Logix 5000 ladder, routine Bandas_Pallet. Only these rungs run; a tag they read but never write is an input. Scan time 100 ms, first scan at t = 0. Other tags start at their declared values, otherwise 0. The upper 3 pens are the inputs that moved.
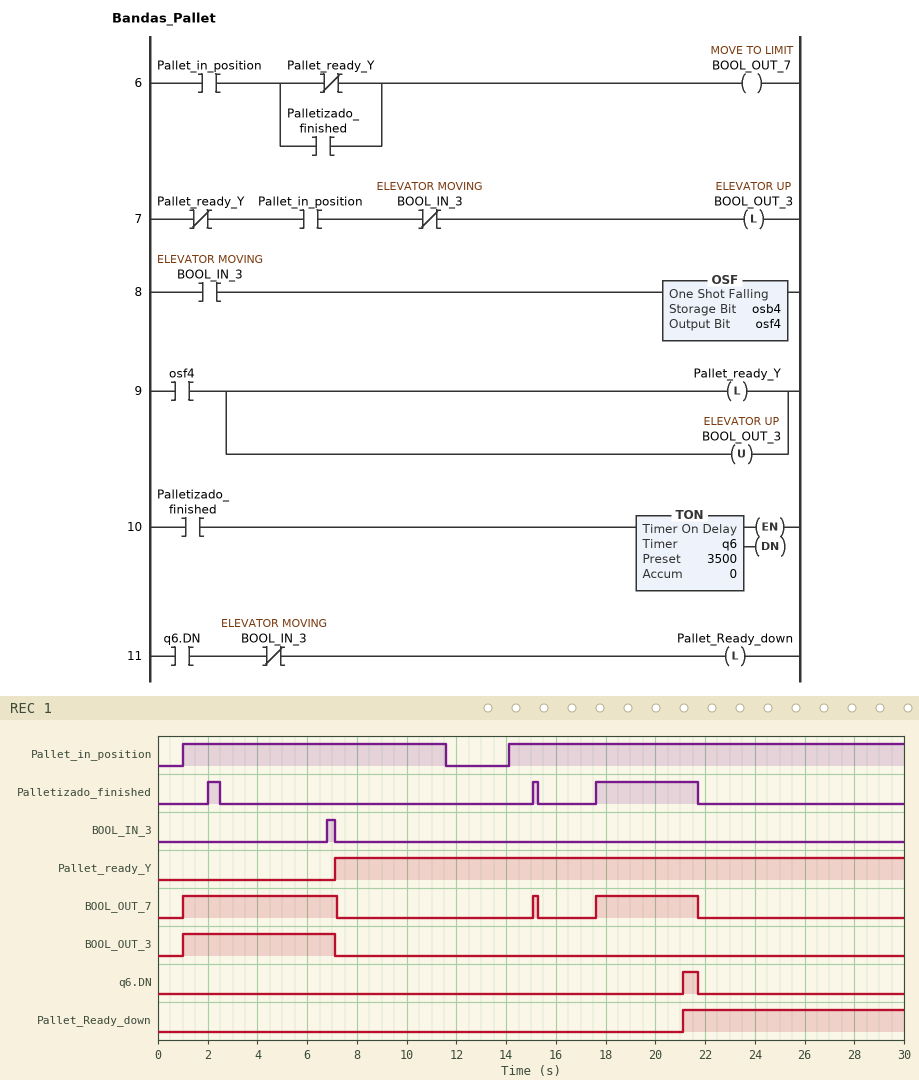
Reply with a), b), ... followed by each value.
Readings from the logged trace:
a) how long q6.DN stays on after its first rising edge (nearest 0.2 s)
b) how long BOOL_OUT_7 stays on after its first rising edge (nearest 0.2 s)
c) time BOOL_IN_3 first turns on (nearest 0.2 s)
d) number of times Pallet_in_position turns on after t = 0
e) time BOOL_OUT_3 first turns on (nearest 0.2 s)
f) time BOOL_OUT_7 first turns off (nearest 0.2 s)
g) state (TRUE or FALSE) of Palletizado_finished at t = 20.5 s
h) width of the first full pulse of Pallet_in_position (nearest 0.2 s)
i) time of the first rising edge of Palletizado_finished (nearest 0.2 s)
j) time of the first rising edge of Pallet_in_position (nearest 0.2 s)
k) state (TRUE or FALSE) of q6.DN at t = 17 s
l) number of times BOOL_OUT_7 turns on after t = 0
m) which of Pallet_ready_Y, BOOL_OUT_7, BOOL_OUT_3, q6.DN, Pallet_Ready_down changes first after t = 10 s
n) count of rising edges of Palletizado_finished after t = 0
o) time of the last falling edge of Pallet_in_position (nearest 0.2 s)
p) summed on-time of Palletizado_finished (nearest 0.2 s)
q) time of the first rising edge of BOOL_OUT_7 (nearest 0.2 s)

a) 0.6 s
b) 6.2 s
c) 6.8 s
d) 2
e) 1.0 s
f) 7.2 s
g) TRUE
h) 10.6 s
i) 2.0 s
j) 1.0 s
k) FALSE
l) 3
m) BOOL_OUT_7
n) 3
o) 11.6 s
p) 4.8 s
q) 1.0 s
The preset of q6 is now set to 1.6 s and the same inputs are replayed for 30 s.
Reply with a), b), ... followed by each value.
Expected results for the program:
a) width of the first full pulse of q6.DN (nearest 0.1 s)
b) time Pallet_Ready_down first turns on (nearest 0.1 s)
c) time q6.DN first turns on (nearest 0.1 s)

a) 2.5 s
b) 19.2 s
c) 19.2 s
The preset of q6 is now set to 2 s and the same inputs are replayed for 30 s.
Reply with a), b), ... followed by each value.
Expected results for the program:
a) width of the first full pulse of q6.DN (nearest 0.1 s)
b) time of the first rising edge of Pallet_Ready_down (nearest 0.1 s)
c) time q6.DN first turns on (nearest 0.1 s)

a) 2.1 s
b) 19.6 s
c) 19.6 s
